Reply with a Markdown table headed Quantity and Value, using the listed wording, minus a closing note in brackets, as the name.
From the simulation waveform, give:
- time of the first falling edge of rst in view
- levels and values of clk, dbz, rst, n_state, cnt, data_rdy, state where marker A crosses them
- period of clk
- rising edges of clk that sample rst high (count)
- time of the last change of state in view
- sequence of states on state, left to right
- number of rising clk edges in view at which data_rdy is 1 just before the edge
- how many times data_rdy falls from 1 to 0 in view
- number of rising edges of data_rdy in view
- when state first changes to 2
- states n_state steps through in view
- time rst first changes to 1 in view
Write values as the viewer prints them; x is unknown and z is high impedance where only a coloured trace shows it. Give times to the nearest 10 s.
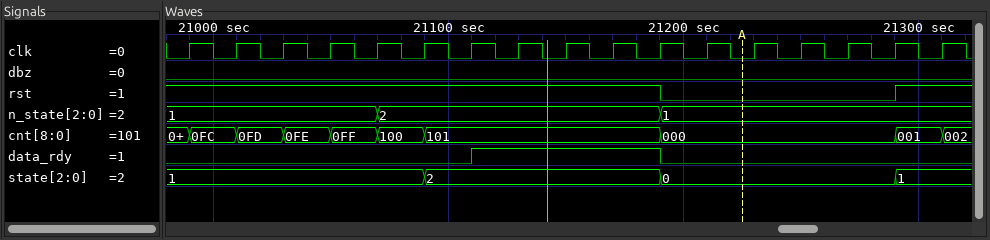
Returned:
| Quantity | Value |
|---|---|
| time of the first falling edge of rst in view | 21190 s |
| levels and values of clk, dbz, rst, n_state, cnt, data_rdy, state where marker A crosses them | clk=0, dbz=0, rst=0, n_state=1, cnt=000, data_rdy=0, state=0 |
| period of clk | 20 s |
| rising edges of clk that sample rst high | 12 |
| time of the last change of state in view | 21290 s |
| sequence of states on state, left to right | 1, 2, 0, 1 |
| number of rising clk edges in view at which data_rdy is 1 just before the edge | 4 |
| how many times data_rdy falls from 1 to 0 in view | 1 |
| number of rising edges of data_rdy in view | 1 |
| when state first changes to 2 | 21090 s |
| states n_state steps through in view | 1, 2, 1 |
| time rst first changes to 1 in view | 21290 s |
